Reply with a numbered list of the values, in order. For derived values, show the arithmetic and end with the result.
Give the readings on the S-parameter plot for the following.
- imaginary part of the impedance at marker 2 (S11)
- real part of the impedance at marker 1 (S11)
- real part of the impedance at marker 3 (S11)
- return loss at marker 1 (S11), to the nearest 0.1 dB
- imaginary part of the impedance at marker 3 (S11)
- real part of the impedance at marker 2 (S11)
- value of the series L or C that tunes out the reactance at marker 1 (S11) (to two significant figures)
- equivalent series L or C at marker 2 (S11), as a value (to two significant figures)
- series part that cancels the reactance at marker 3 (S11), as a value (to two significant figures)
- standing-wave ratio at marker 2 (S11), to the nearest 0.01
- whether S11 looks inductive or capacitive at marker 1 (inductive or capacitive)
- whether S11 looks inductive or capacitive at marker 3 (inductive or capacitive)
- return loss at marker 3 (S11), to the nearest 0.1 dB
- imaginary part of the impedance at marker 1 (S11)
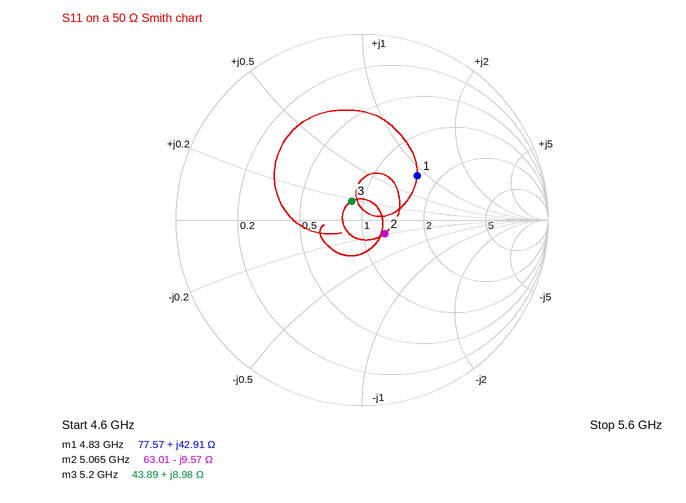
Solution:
1. -9.57 Ω
2. 77.57 Ω
3. 43.89 Ω
4. 8.4 dB
5. +8.98 Ω
6. 63.01 Ω
7. C = 1/(2π × 4.83 GHz × 42.91 Ω) ≈ 768 fF, so 770 fF to two significant figures
8. C = 1/(2π × 5.065 GHz × 9.57 Ω) ≈ 3.3 pF
9. C = 1/(2π × 5.2 GHz × 8.98 Ω) ≈ 3.4 pF
10. 1.33
11. inductive
12. inductive
13. 18.8 dB
14. +42.91 Ω
